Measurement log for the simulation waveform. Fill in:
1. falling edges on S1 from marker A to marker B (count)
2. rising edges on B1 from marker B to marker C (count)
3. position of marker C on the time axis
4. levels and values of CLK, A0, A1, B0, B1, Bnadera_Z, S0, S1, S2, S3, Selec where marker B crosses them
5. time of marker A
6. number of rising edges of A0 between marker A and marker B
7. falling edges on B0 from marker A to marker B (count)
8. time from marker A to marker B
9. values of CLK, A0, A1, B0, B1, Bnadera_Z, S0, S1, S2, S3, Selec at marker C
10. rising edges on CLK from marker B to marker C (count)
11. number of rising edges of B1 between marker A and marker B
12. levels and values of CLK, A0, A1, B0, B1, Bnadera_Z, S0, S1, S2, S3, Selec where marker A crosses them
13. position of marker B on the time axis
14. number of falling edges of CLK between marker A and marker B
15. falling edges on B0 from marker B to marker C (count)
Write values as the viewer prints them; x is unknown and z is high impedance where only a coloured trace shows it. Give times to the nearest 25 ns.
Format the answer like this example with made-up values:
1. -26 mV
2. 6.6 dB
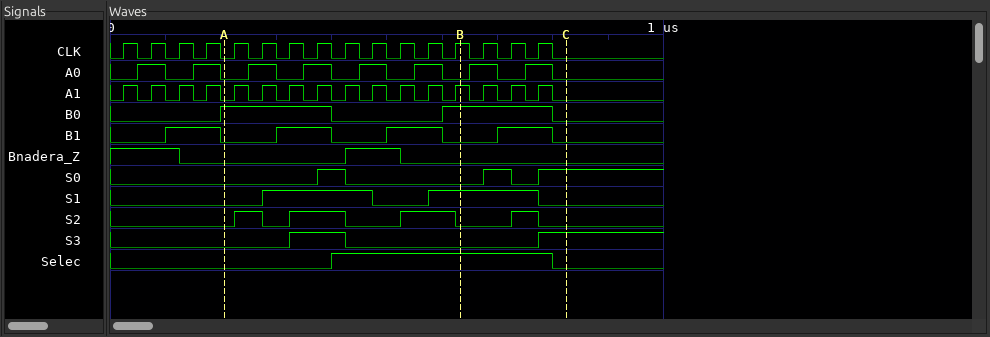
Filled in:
1. 1
2. 1
3. 825 ns
4. CLK=1, A0=0, A1=1, B0=1, B1=0, Bnadera_Z=0, S0=0, S1=1, S2=0, S3=0, Selec=1
5. 200 ns
6. 4
7. 1
8. 425 ns
9. CLK=0, A0=0, A1=0, B0=0, B1=0, Bnadera_Z=0, S0=1, S1=0, S2=0, S3=1, Selec=0
10. 3
11. 2
12. CLK=0, A0=0, A1=0, B0=1, B1=0, Bnadera_Z=0, S0=0, S1=0, S2=0, S3=0, Selec=0
13. 625 ns
14. 8
15. 1
